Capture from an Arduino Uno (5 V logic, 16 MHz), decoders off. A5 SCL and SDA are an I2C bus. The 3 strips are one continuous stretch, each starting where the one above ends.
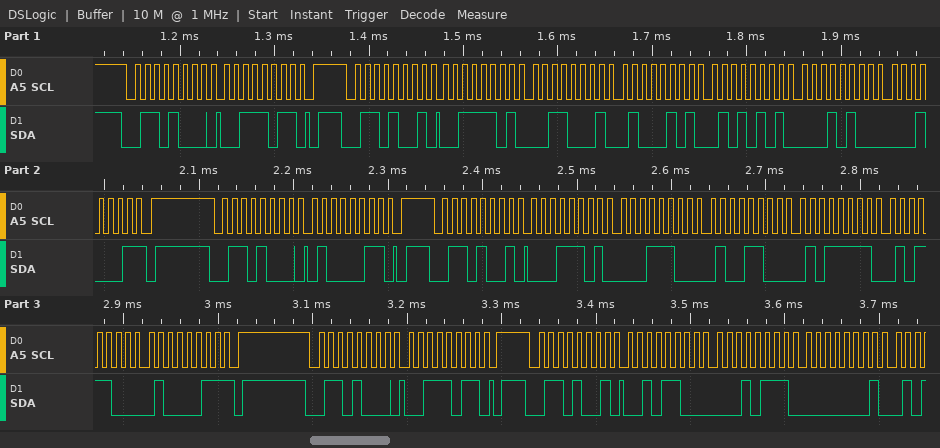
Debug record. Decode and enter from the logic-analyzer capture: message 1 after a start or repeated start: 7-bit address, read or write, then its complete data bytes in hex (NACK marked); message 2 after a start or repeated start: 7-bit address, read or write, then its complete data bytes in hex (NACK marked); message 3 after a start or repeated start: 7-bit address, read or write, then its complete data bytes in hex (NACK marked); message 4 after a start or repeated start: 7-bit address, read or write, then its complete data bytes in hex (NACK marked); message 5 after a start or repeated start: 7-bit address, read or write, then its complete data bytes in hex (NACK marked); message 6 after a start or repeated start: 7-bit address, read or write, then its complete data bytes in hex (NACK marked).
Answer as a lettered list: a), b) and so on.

a) 0x34 write: 3B
b) 0x34 read: 3D 31 45 55 14 11 NACK
c) 0x34 write: 43
d) 0x34 read: 1D 1C 4C 5F 5C 43 NACK
e) 0x34 write: 3B
f) 0x34 read: 2C 17 01
